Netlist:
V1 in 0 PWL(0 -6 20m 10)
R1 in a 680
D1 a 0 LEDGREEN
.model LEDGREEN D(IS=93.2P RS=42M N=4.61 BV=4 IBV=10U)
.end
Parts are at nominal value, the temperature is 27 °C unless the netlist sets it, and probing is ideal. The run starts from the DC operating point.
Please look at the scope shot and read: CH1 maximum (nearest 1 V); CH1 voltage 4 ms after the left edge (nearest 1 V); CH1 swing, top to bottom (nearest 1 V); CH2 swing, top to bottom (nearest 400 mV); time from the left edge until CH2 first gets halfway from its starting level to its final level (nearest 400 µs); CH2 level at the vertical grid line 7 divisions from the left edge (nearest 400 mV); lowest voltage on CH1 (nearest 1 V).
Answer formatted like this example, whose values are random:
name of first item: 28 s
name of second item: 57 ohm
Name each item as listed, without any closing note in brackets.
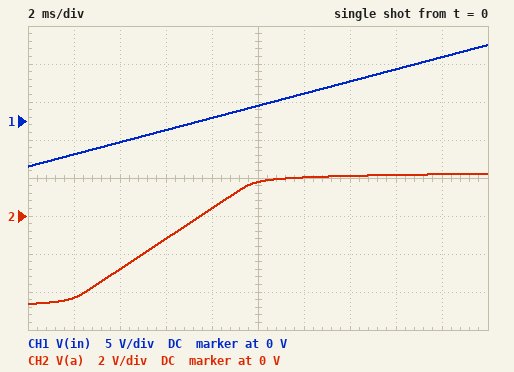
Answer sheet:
CH1 maximum: 10 V
CH1 voltage 4 ms after the left edge: -3 V
CH1 swing, top to bottom: 16 V
CH2 swing, top to bottom: 6.8 V
time from the left edge until CH2 first gets halfway from its starting level to its final level: 6.0 ms
CH2 level at the vertical grid line 7 divisions from the left edge: 2.0 V
lowest voltage on CH1: -6 V
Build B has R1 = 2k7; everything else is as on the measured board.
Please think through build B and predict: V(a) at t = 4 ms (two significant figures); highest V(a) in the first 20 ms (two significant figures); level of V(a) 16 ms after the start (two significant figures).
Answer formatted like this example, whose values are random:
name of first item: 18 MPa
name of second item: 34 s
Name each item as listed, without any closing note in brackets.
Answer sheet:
V(a) at t = 4 ms: -2.8 V
highest V(a) in the first 20 ms: 2.1 V
level of V(a) 16 ms after the start: 2.0 V
